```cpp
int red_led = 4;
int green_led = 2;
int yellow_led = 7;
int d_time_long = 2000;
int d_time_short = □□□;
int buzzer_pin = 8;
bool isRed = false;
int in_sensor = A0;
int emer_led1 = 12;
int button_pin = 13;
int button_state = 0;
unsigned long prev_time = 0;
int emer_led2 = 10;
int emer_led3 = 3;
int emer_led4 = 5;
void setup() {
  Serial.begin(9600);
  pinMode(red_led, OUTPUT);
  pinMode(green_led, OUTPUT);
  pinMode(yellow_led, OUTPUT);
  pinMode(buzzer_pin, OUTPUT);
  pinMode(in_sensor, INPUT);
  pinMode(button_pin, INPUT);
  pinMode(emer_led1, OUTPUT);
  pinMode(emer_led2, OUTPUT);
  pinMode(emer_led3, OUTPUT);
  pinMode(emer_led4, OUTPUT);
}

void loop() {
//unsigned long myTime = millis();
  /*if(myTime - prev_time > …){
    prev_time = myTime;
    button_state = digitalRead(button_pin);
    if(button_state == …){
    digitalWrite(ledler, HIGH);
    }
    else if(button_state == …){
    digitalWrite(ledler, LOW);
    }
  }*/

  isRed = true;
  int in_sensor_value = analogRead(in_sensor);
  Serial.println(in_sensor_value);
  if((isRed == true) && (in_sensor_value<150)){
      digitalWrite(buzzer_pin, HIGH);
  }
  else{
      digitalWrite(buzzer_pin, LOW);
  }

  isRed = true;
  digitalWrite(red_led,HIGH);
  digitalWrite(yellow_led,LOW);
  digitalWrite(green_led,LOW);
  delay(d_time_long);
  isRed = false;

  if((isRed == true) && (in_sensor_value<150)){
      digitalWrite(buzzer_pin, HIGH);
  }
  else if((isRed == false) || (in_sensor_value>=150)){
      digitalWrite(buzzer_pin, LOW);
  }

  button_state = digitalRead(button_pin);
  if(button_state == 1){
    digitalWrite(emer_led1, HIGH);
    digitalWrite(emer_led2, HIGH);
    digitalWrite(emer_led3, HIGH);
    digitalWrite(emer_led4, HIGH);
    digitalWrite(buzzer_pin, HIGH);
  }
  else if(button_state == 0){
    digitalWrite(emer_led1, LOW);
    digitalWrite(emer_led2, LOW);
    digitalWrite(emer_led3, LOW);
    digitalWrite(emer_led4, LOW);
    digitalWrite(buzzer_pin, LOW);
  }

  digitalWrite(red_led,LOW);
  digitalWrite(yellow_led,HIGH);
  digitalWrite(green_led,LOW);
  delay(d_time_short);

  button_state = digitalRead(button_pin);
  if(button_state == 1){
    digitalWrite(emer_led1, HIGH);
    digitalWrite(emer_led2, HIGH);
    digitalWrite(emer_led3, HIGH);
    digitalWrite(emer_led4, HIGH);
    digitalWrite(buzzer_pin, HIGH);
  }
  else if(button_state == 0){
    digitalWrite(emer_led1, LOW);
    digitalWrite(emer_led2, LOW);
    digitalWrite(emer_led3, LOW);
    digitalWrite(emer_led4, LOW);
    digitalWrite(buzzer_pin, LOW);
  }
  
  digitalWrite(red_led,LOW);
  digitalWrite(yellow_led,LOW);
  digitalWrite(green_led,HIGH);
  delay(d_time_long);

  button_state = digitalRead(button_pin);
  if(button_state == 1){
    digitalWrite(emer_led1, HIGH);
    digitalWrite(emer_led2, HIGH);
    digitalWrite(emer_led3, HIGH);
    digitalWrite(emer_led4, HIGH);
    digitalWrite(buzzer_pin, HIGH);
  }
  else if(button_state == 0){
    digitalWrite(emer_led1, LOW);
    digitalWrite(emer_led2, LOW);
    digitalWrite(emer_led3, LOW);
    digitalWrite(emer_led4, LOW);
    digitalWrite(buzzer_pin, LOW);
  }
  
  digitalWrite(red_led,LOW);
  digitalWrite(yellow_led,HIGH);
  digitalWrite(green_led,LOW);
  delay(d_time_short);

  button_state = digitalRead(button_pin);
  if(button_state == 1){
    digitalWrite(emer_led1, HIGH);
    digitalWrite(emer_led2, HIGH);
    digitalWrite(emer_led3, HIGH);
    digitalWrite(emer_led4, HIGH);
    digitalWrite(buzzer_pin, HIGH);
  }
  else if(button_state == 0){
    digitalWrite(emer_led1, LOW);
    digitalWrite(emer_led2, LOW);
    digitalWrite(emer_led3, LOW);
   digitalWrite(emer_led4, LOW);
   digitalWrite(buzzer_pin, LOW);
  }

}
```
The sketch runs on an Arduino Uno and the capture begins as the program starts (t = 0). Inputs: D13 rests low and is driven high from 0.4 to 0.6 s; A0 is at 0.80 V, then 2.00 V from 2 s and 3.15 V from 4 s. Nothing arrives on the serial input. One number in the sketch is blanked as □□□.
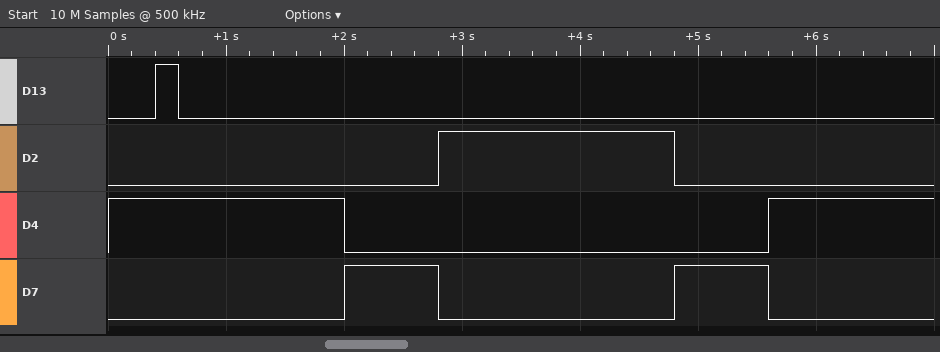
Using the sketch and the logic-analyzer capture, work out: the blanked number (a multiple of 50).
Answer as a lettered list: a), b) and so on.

a) 800
